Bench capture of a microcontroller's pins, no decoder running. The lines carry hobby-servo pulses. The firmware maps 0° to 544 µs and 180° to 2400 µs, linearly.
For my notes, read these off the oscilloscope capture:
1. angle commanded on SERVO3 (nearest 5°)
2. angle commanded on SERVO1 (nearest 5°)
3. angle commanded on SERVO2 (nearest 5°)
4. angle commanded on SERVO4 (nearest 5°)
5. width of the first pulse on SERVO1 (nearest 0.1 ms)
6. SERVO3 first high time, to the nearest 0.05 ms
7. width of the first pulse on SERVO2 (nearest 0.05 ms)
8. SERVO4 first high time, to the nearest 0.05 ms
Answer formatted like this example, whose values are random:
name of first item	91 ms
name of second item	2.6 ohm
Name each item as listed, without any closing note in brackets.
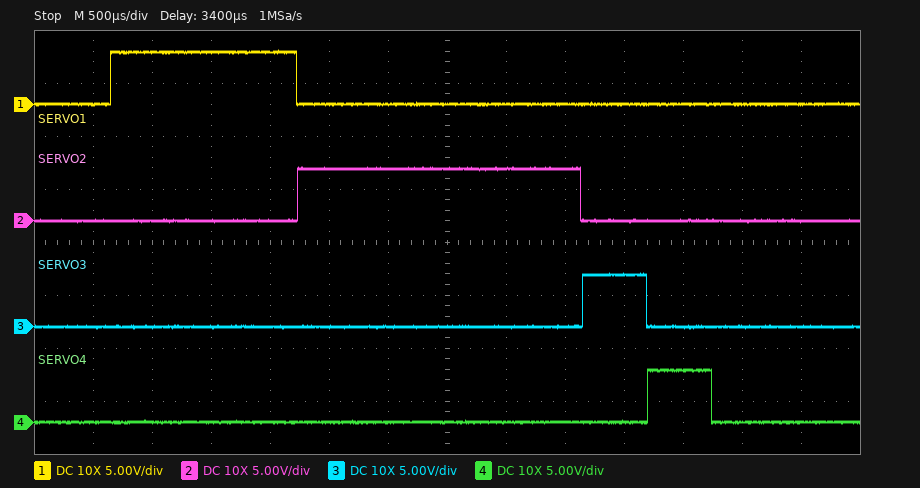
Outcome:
angle commanded on SERVO3	0°
angle commanded on SERVO1	100°
angle commanded on SERVO2	180°
angle commanded on SERVO4	0°
width of the first pulse on SERVO1	1.6 ms
SERVO3 first high time, to the nearest 0.05 ms	0.55 ms
width of the first pulse on SERVO2	2.40 ms
SERVO4 first high time, to the nearest 0.05 ms	0.55 ms
